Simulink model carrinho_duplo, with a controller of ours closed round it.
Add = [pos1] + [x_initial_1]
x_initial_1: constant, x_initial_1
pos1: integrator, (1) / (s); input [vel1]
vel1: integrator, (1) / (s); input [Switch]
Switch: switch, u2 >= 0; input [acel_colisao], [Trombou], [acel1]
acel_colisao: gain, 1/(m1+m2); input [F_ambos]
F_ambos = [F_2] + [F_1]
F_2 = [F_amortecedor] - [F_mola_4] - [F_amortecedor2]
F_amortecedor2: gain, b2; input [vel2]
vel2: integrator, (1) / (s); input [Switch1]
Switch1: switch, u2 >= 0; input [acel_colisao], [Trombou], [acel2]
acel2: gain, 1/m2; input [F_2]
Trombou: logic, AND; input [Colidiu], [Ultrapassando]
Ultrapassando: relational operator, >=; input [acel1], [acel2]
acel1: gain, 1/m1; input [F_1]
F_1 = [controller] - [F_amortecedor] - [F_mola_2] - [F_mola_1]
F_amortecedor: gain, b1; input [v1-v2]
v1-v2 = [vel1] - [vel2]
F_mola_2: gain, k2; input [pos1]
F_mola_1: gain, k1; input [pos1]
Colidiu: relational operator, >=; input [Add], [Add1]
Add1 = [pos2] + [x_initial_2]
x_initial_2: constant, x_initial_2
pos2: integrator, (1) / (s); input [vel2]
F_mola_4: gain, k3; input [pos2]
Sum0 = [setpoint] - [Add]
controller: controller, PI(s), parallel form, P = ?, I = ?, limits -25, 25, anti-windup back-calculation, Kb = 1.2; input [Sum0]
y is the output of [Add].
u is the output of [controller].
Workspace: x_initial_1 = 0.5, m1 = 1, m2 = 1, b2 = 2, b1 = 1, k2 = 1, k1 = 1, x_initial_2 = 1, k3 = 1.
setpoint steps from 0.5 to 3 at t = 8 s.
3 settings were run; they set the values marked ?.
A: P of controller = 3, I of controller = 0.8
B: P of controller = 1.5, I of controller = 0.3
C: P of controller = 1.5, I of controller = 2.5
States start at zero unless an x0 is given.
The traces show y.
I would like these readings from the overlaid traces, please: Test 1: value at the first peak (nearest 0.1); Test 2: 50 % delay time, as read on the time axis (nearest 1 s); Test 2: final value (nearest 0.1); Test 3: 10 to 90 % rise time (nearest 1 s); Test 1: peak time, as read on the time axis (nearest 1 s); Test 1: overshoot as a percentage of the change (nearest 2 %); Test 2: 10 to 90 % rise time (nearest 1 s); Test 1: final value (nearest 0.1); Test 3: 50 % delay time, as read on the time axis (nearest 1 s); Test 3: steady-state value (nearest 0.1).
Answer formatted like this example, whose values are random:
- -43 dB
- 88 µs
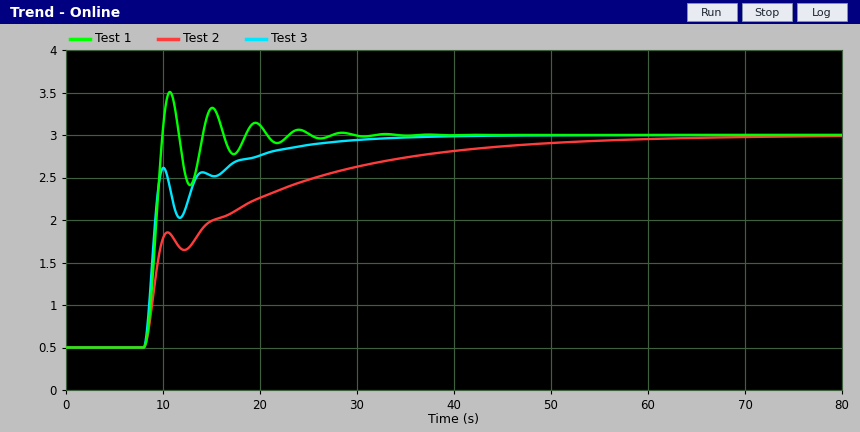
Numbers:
- 3.5
- 10 s
- 3.0
- 11 s
- 11 s
- 20 %
- 27 s
- 3.0
- 9 s
- 3.0
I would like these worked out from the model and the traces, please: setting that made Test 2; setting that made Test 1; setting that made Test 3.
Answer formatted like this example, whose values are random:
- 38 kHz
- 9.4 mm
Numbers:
- B
- C
- A
